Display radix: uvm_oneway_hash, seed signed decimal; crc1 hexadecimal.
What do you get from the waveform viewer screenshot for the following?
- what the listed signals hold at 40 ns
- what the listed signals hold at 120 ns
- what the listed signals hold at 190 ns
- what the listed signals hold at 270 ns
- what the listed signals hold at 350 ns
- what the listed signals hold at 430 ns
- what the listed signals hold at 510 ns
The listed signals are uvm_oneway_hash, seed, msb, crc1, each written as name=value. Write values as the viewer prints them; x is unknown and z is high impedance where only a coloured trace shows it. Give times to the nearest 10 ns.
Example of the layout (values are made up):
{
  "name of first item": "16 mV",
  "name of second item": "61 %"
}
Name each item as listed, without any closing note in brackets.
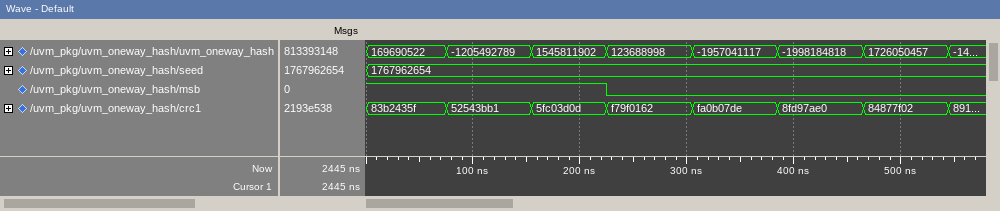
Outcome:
{
  "what the listed signals hold at 40 ns": "uvm_oneway_hash=169690522, seed=1767962654, msb=1, crc1=83b2435f",
  "what the listed signals hold at 120 ns": "uvm_oneway_hash=-1205492789, seed=1767962654, msb=1, crc1=52543bb1",
  "what the listed signals hold at 190 ns": "uvm_oneway_hash=1545811902, seed=1767962654, msb=1, crc1=5fc03d0d",
  "what the listed signals hold at 270 ns": "uvm_oneway_hash=123688998, seed=1767962654, msb=0, crc1=f79f0162",
  "what the listed signals hold at 350 ns": "uvm_oneway_hash=-1957041117, seed=1767962654, msb=0, crc1=fa0b07de",
  "what the listed signals hold at 430 ns": "uvm_oneway_hash=-1998184818, seed=1767962654, msb=0, crc1=8fd97ae0",
  "what the listed signals hold at 510 ns": "uvm_oneway_hash=1726050457, seed=1767962654, msb=0, crc1=84877f02"
}
